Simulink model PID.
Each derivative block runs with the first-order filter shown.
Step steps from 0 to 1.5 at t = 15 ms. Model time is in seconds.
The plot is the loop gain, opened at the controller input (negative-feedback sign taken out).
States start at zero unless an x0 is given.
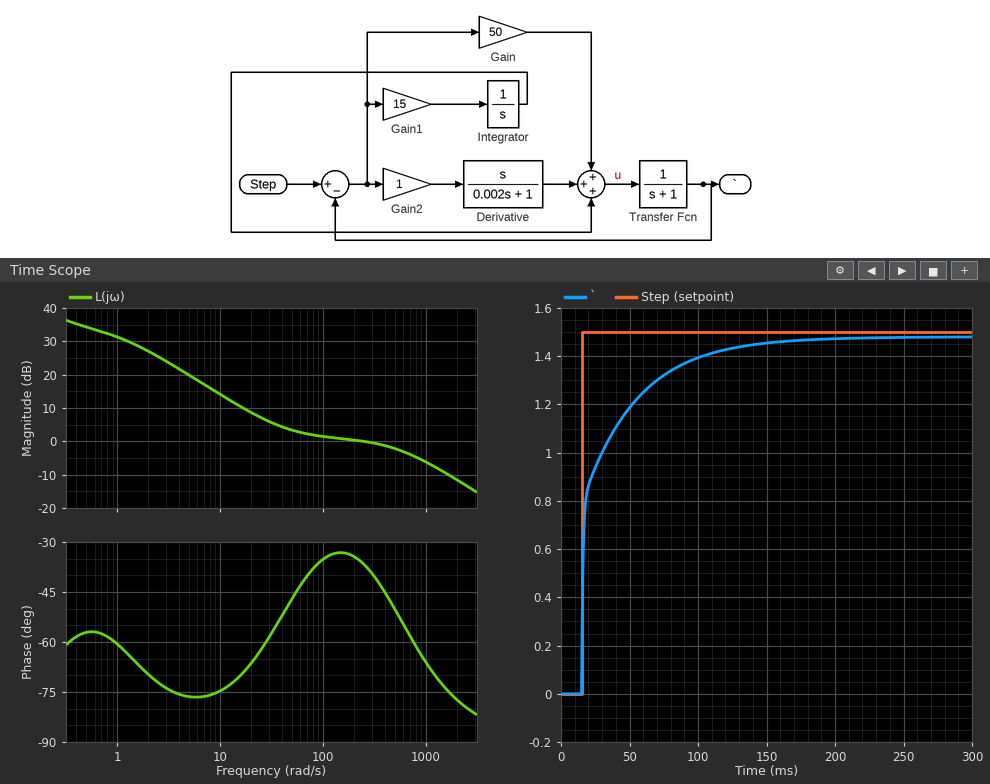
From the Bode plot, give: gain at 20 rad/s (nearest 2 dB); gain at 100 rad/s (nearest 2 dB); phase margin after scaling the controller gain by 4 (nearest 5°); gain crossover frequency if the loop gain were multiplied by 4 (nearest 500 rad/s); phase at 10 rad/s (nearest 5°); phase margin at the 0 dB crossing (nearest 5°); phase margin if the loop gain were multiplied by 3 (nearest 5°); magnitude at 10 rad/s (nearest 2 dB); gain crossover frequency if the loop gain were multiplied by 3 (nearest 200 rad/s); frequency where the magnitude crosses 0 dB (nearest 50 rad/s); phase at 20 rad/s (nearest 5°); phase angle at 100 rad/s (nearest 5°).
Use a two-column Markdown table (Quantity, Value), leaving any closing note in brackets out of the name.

| Quantity | Value |
|---|---|
| gain at 20 rad/s | 8 dB |
| gain at 100 rad/s | 2 dB |
| phase margin after scaling the controller gain by 4 | 100° |
| gain crossover frequency if the loop gain were multiplied by 4 | 2000 rad/s |
| phase at 10 rad/s | -75° |
| phase margin at the 0 dB crossing | 145° |
| phase margin if the loop gain were multiplied by 3 | 105° |
| magnitude at 10 rad/s | 14 dB |
| gain crossover frequency if the loop gain were multiplied by 3 | 1600 rad/s |
| frequency where the magnitude crosses 0 dB | 250 rad/s |
| phase at 20 rad/s | -65° |
| phase angle at 100 rad/s | -35° |
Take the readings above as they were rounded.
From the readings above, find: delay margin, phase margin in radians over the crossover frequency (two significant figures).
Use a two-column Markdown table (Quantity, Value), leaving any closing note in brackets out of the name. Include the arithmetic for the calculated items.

| Quantity | Value |
|---|---|
| delay margin, phase margin in radians over the crossover frequency | 145 × π / 180 / 250 = 0.010 s |
